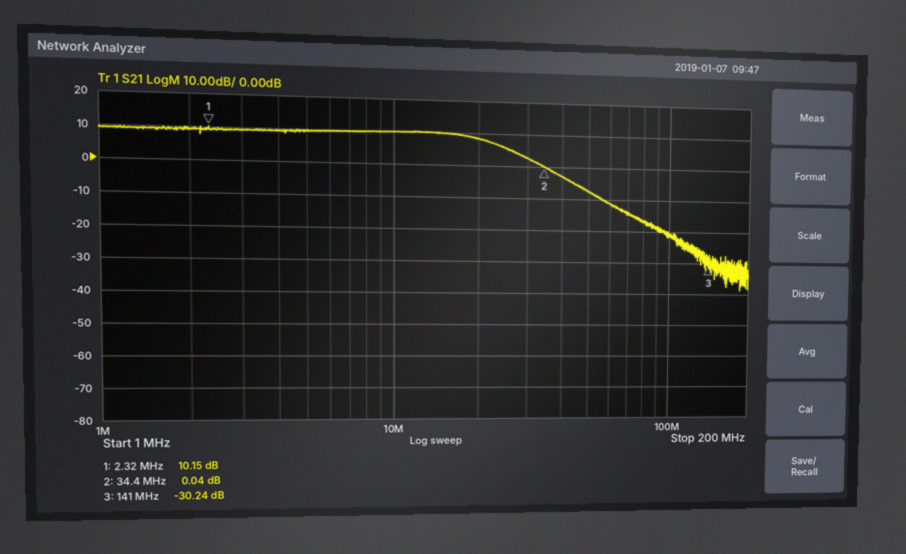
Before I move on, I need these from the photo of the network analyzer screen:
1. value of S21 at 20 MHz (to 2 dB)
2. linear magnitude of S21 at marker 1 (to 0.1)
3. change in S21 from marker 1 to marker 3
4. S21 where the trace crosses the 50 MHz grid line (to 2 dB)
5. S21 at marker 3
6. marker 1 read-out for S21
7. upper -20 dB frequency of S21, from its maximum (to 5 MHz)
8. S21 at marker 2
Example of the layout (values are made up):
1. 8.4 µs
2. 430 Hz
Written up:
1. 8 dB
2. 3.2
3. -40.39 dB
4. -8 dB
5. -30.24 dB
6. 10.15 dB
7. 55 MHz
8. 0.04 dB
